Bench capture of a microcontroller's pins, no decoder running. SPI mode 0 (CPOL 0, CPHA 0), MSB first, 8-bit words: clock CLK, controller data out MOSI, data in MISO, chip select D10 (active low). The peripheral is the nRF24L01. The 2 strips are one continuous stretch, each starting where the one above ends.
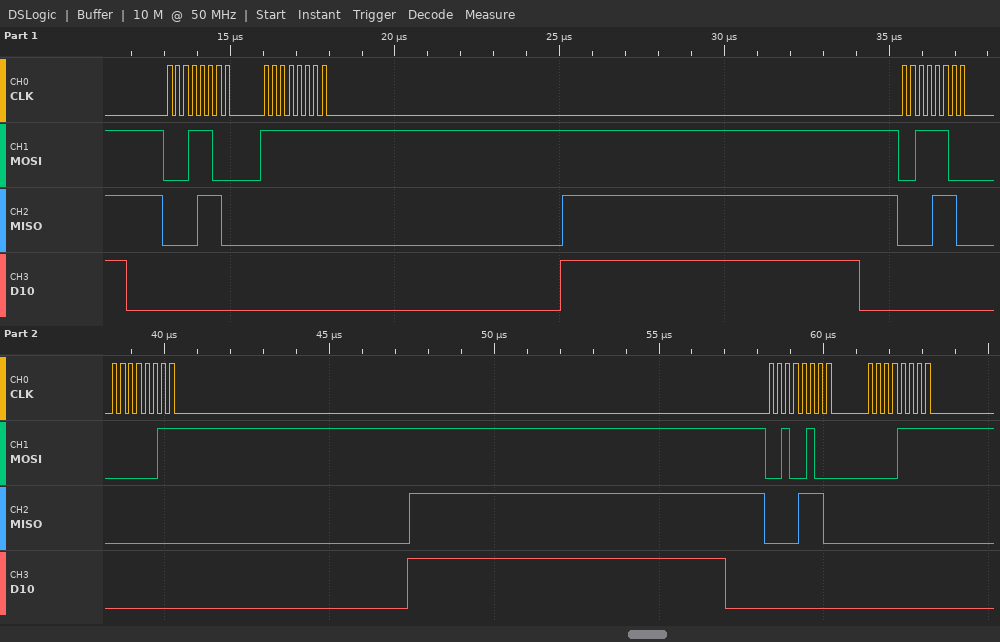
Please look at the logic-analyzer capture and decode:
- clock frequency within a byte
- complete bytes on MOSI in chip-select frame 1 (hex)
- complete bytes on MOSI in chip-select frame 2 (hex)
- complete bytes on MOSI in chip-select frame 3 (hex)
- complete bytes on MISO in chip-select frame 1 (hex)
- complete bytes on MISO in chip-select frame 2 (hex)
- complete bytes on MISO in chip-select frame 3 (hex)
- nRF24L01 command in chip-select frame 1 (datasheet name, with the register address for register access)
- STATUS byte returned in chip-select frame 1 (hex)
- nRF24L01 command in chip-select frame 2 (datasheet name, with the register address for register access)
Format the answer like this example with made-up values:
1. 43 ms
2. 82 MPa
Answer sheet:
1. 4 MHz
2. 1C FF
3. 3C 03
4. 24 0F
5. 0E 00
6. 0E 00
7. 0E 00
8. R_REGISTER 0x1C
9. 0x0E
10. W_REGISTER 0x1C
